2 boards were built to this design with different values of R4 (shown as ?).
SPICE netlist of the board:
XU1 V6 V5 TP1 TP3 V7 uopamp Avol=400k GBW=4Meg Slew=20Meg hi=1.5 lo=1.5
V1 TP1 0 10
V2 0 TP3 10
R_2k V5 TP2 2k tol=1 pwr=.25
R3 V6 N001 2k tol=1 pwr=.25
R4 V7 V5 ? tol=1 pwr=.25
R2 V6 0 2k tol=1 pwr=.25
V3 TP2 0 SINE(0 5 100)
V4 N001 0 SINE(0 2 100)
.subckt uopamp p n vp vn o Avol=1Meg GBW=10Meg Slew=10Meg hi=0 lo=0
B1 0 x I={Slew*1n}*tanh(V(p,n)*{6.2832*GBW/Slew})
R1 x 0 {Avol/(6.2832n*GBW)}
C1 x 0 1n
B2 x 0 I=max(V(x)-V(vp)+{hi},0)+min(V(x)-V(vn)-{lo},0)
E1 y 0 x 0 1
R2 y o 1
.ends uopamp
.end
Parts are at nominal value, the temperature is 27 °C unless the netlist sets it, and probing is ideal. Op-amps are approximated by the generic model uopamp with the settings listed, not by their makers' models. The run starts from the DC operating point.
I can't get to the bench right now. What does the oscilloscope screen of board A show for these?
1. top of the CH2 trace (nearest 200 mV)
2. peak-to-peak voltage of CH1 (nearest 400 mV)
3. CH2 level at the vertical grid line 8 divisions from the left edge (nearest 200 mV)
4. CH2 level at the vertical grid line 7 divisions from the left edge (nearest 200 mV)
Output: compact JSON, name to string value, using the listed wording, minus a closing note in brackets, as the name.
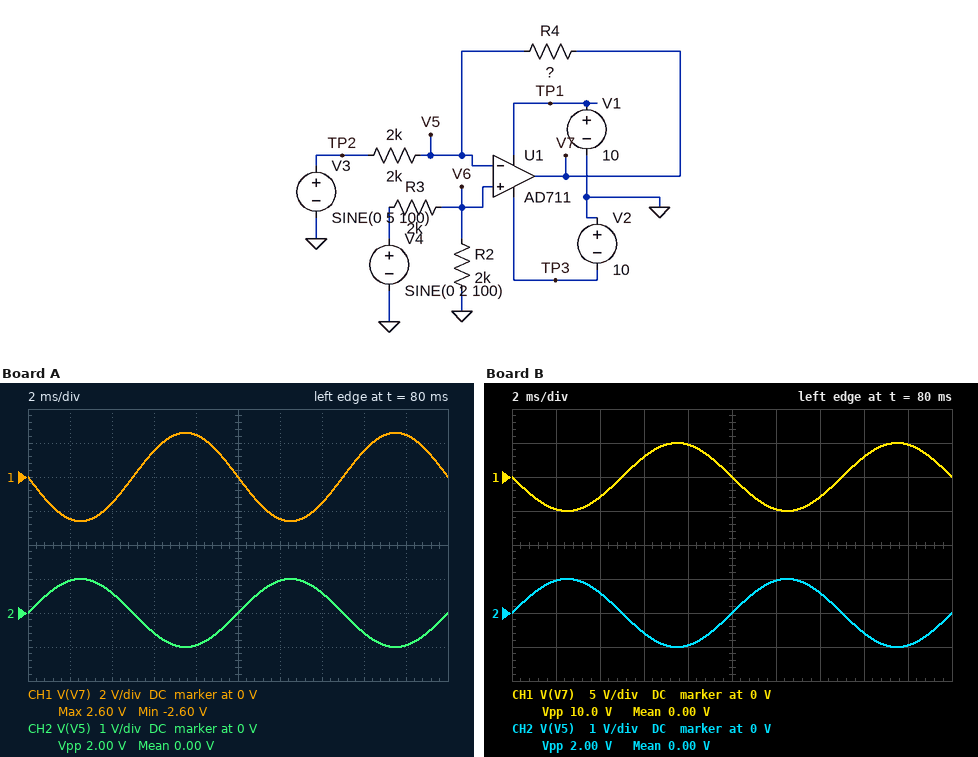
{"top of the CH2 trace": "1.0 V", "peak-to-peak voltage of CH1": "5.2 V", "CH2 level at the vertical grid line 8 divisions from the left edge": "-600 mV", "CH2 level at the vertical grid line 7 divisions from the left edge": "600 mV"}
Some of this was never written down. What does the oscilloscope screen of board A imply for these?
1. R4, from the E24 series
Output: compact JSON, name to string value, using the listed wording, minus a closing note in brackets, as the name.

{"R4, from the E24 series": "1.8 kΩ"}
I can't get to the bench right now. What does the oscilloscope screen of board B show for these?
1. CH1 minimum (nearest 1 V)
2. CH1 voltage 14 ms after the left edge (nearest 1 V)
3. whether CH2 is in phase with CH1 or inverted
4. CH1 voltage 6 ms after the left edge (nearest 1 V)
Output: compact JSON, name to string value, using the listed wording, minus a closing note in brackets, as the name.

{"CH1 minimum": "-5 V", "CH1 voltage 14 ms after the left edge": "-3 V", "whether CH2 is in phase with CH1 or inverted": "inverted", "CH1 voltage 6 ms after the left edge": "3 V"}
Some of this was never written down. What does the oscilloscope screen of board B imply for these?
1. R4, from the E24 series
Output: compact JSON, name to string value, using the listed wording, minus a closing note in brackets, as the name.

{"R4, from the E24 series": "3 kΩ"}
